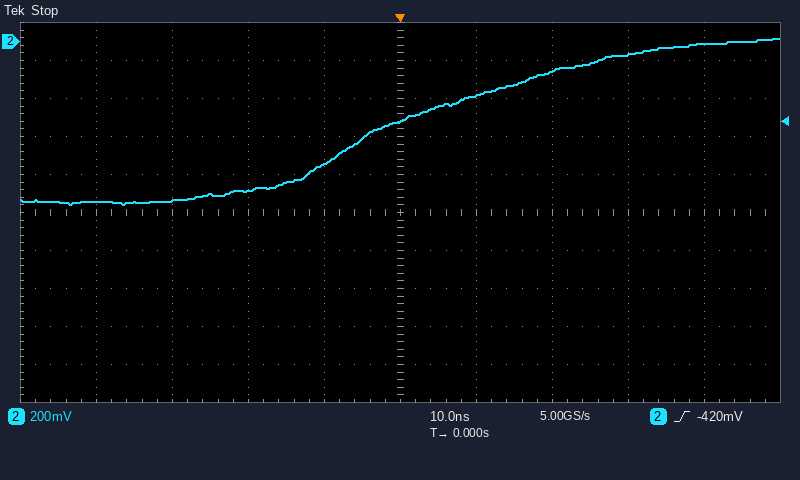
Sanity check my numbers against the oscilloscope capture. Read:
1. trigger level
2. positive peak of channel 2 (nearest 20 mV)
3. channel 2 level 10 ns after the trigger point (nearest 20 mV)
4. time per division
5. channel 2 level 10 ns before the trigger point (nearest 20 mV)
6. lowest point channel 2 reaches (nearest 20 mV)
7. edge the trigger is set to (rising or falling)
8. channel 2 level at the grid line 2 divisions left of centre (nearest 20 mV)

-420 mV
20 mV
-280 mV
10 ns
-640 mV
-860 mV
rising
-780 mV
